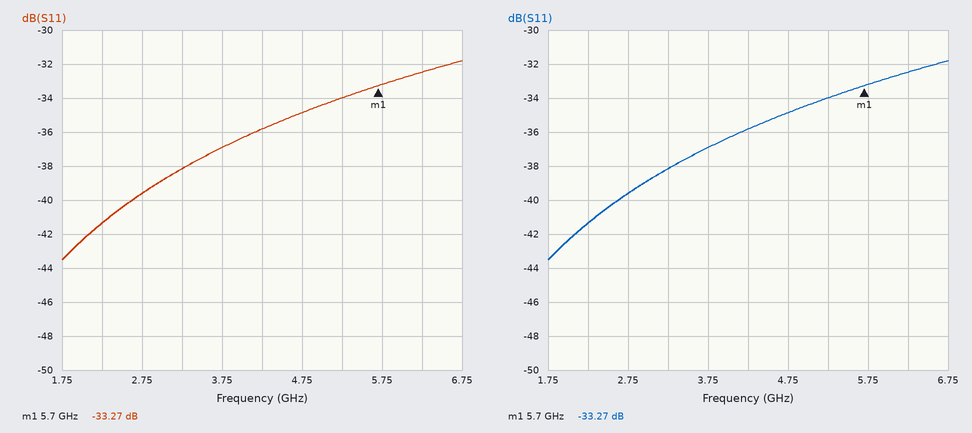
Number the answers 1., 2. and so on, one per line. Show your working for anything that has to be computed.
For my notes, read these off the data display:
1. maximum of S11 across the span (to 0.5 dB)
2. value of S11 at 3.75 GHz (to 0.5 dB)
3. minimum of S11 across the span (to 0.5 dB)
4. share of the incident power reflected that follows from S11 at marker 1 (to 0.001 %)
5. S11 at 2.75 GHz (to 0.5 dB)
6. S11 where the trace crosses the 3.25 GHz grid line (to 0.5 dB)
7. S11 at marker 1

1. -32.0 dB
2. -37.0 dB
3. -43.5 dB
4. 10^(-33.27/10) ≈ 0.047 %
5. -39.5 dB
6. -38.0 dB
7. -33.27 dB
